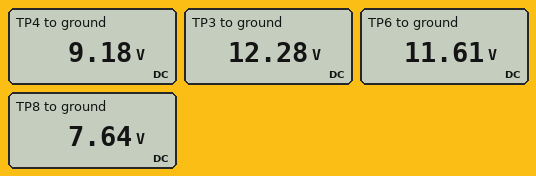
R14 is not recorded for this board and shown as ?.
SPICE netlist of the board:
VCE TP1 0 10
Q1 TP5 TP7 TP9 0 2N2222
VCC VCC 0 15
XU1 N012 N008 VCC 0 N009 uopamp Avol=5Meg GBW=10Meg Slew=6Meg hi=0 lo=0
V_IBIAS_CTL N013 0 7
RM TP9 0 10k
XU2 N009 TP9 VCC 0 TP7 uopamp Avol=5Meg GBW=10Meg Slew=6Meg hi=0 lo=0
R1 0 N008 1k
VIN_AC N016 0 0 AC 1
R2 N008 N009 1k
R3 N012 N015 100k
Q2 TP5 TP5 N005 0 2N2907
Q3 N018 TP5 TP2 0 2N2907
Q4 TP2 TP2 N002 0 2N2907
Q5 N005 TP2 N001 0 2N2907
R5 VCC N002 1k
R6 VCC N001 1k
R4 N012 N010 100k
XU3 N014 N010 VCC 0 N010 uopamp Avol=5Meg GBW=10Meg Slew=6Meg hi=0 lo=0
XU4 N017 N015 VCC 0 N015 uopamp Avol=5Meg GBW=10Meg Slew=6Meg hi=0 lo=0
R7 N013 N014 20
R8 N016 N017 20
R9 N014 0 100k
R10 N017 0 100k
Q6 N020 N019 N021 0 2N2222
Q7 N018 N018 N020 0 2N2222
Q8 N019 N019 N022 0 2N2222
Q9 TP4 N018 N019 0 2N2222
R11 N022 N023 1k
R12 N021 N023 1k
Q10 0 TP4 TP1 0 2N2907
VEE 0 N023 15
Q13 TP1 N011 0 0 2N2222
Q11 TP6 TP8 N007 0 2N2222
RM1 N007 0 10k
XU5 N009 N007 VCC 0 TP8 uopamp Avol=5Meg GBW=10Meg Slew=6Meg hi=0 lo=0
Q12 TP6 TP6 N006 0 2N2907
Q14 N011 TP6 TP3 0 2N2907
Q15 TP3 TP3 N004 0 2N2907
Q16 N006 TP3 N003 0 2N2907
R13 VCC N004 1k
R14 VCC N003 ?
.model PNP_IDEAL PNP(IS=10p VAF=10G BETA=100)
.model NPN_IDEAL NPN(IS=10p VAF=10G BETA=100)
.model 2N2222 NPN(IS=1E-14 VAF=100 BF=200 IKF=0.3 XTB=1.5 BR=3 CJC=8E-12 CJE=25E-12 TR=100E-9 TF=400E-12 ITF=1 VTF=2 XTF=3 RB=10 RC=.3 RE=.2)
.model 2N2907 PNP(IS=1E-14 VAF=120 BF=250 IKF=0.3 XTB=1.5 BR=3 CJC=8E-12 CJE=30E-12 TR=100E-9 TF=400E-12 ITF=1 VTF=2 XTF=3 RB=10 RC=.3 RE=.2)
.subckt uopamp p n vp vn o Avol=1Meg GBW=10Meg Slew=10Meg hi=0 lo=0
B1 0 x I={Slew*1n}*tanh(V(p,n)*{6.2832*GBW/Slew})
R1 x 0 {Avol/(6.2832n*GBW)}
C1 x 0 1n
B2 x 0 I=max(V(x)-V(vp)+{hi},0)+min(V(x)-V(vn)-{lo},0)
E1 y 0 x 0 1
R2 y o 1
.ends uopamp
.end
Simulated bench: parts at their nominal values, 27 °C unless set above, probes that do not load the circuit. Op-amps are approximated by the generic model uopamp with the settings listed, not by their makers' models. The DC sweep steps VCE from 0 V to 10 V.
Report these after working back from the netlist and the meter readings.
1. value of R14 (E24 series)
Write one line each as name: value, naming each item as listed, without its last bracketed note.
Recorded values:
value of R14: 3 kΩ
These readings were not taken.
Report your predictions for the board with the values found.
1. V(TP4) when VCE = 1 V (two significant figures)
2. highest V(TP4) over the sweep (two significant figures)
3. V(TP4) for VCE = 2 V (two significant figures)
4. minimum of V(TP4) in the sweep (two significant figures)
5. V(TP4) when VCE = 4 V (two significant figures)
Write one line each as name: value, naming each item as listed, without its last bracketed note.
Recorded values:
V(TP4) when VCE = 1 V: 180 mV
highest V(TP4) over the sweep: 9.2 V
V(TP4) for VCE = 2 V: 1.2 V
minimum of V(TP4) in the sweep: -680 mV
V(TP4) when VCE = 4 V: 3.2 V
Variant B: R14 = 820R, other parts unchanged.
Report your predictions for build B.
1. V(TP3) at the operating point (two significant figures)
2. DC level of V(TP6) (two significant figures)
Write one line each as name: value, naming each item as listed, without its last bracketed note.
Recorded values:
V(TP3) at the operating point: 14 V
DC level of V(TP6): 13 V
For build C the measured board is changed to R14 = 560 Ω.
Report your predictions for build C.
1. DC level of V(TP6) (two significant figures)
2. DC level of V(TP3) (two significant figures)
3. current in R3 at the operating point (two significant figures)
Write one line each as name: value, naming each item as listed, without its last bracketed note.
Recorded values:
DC level of V(TP6): 13 V
DC level of V(TP3): 14 V
current in R3 at the operating point: 35 µA
